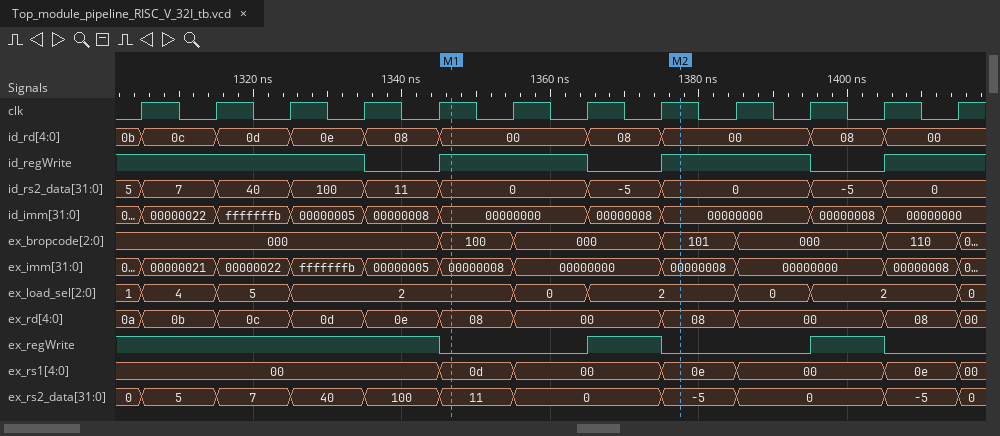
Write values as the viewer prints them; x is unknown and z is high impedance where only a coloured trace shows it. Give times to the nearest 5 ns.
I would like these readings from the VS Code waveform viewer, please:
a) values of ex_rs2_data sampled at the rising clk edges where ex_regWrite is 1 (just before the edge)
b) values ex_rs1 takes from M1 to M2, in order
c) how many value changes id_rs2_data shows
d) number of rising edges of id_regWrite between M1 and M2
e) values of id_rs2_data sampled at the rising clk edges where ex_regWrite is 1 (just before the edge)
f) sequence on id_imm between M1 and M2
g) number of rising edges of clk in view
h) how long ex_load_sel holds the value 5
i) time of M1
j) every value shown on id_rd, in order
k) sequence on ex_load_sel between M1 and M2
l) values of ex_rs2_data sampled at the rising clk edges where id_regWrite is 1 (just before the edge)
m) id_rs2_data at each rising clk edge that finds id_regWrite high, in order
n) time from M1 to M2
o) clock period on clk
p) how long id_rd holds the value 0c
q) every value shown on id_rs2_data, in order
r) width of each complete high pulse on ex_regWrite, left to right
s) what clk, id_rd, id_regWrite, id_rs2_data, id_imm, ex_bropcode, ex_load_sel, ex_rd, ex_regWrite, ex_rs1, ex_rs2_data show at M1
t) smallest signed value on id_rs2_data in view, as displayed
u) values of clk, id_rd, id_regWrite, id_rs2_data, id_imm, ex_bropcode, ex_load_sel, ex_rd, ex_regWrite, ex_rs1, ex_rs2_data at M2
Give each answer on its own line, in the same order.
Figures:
0, 5, 7, 40, 100, 0, 0
0d, 00, 0e
9
1
5, 7, 40, 100, 11, -5, -5
00000000, 00000008, 00000000
12
10 ns
1345 ns
0b, 0c, 0d, 0e, 08, 00, 08, 00, 08, 00
2, 0, 2
0, 5, 7, 40, 11, 0, -5, 0, -5
5, 7, 40, 100, 0, 0, 0, 0, 0
30 ns
10 ns
10 ns
5, 7, 40, 100, 11, 0, -5, 0, -5, 0
10 ns, 10 ns
clk=1, id_rd=00, id_regWrite=1, id_rs2_data=0, id_imm=00000000, ex_bropcode=100, ex_load_sel=2, ex_rd=08, ex_regWrite=0, ex_rs1=0d, ex_rs2_data=11
-5
clk=1, id_rd=00, id_regWrite=1, id_rs2_data=0, id_imm=00000000, ex_bropcode=101, ex_load_sel=2, ex_rd=08, ex_regWrite=0, ex_rs1=0e, ex_rs2_data=-5
